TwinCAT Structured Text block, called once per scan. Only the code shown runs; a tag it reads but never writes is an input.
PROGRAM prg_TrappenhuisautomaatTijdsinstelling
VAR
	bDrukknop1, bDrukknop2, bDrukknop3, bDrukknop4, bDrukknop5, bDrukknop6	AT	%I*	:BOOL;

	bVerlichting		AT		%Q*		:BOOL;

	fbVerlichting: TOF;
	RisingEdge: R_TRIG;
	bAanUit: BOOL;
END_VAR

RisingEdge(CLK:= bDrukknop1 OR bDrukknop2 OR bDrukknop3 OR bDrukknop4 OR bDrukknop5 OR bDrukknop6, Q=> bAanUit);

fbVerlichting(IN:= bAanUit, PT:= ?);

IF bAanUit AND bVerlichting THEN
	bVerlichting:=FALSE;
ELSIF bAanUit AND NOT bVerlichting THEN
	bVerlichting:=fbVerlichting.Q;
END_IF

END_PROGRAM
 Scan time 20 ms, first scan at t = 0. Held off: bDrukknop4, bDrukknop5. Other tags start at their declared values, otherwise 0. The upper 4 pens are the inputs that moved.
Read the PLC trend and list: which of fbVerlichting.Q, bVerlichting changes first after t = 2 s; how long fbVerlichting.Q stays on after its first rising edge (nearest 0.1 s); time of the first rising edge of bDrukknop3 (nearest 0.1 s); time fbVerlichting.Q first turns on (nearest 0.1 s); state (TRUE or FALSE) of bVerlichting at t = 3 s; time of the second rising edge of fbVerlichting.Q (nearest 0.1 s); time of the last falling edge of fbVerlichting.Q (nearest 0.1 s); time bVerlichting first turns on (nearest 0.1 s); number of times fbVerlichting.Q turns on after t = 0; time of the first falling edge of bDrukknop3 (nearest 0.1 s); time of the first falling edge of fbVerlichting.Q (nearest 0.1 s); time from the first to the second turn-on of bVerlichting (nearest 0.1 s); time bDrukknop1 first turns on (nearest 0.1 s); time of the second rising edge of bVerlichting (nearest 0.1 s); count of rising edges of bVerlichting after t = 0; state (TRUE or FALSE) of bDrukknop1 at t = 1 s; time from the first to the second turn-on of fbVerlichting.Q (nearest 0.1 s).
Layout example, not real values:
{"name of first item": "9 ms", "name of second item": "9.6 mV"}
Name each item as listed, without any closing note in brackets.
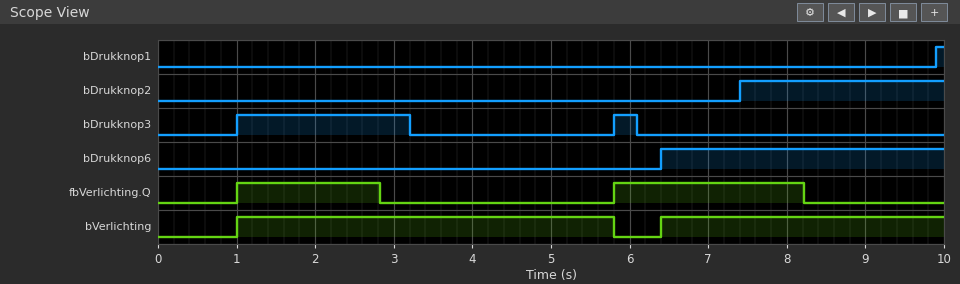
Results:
{"which of fbVerlichting.Q, bVerlichting changes first after t = 2 s": "fbVerlichting.Q", "how long fbVerlichting.Q stays on after its first rising edge": "1.8 s", "time of the first rising edge of bDrukknop3": "1.0 s", "time fbVerlichting.Q first turns on": "1.0 s", "state (TRUE or FALSE) of bVerlichting at t = 3 s": "TRUE", "time of the second rising edge of fbVerlichting.Q": "5.8 s", "time of the last falling edge of fbVerlichting.Q": "8.2 s", "time bVerlichting first turns on": "1.0 s", "number of times fbVerlichting.Q turns on after t = 0": "2", "time of the first falling edge of bDrukknop3": "3.2 s", "time of the first falling edge of fbVerlichting.Q": "2.8 s", "time from the first to the second turn-on of bVerlichting": "5.4 s", "time bDrukknop1 first turns on": "9.9 s", "time of the second rising edge of bVerlichting": "6.4 s", "count of rising edges of bVerlichting after t = 0": "2", "state (TRUE or FALSE) of bDrukknop1 at t = 1 s": "FALSE", "time from the first to the second turn-on of fbVerlichting.Q": "4.8 s"}
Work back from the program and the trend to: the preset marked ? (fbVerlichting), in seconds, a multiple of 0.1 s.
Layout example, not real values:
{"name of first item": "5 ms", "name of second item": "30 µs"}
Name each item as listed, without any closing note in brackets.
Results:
{"the preset marked ? (fbVerlichting), in seconds, a multiple of 0.1 s": "1.8 s"}
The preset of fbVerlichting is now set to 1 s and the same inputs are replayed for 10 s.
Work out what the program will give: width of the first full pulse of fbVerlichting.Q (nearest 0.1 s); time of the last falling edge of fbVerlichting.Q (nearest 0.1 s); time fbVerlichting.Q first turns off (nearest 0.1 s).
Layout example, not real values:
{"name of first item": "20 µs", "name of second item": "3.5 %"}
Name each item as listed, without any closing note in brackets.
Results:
{"width of the first full pulse of fbVerlichting.Q": "1.0 s", "time of the last falling edge of fbVerlichting.Q": "7.4 s", "time fbVerlichting.Q first turns off": "2.0 s"}
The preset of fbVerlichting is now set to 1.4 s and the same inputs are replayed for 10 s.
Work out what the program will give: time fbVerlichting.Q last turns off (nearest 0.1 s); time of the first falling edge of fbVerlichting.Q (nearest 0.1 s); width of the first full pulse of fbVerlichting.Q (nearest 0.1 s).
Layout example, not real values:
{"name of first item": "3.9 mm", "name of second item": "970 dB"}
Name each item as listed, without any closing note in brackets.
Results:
{"time fbVerlichting.Q last turns off": "7.8 s", "time of the first falling edge of fbVerlichting.Q": "2.4 s", "width of the first full pulse of fbVerlichting.Q": "1.4 s"}
